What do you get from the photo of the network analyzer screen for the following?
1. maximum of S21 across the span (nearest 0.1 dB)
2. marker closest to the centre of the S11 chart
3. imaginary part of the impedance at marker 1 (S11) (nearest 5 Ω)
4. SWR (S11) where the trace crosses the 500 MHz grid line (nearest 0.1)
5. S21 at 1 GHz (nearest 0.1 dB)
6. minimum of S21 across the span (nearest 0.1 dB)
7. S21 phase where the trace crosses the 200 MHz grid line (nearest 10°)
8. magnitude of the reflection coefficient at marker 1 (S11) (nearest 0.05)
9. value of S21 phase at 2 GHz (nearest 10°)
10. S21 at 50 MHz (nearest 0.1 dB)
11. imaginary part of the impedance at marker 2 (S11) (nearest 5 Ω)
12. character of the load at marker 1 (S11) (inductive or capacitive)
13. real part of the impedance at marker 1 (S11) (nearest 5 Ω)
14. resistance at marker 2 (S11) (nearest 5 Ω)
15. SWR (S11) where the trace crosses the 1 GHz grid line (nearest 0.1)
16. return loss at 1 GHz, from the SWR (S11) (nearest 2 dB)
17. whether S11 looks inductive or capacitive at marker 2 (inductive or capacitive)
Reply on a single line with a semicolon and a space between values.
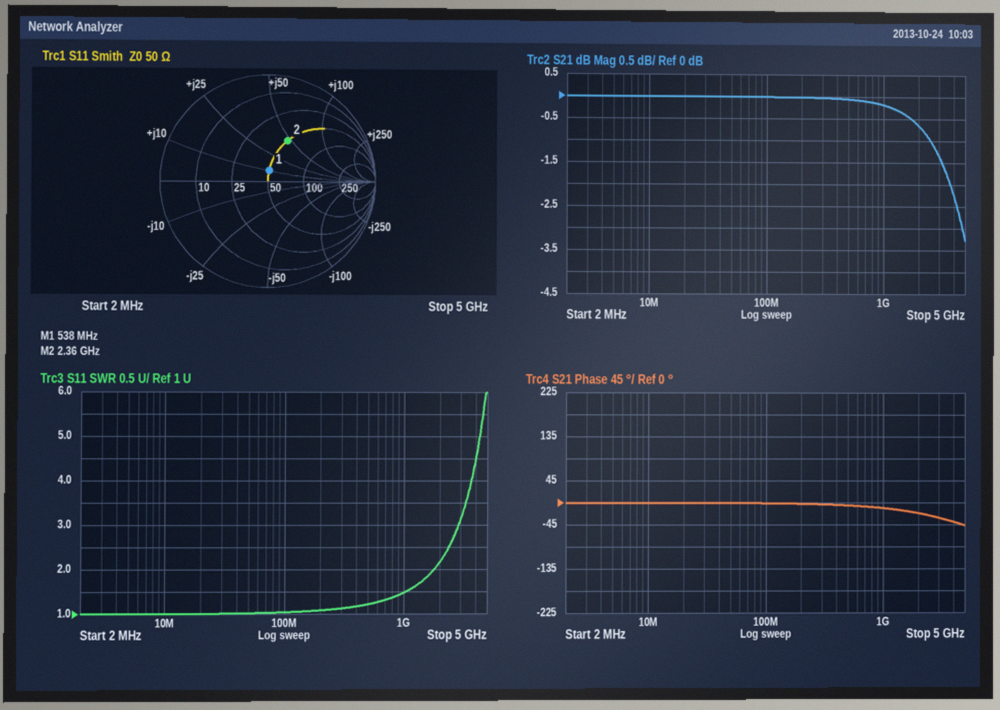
0.0 dB; marker 1; +10 Ω; 1.2; -0.2 dB; -3.3 dB; 0°; 0.10; -20°; 0.0 dB; +45 Ω; inductive; 50 Ω; 50 Ω; 1.5; 14 dB; inductive
